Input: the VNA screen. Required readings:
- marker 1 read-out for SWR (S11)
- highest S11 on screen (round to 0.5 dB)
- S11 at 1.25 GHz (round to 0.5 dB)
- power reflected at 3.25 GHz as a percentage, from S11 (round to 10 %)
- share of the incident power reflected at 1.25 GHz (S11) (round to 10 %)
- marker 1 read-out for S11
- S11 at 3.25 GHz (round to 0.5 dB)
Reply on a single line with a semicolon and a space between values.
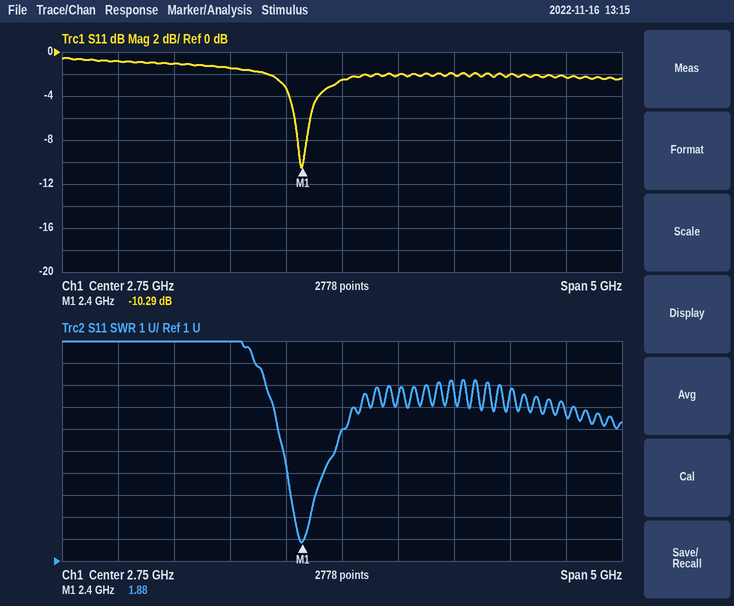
1.88; -0.5 dB; -1.0 dB; 60 %; 80 %; -10.29 dB; -2.0 dB
